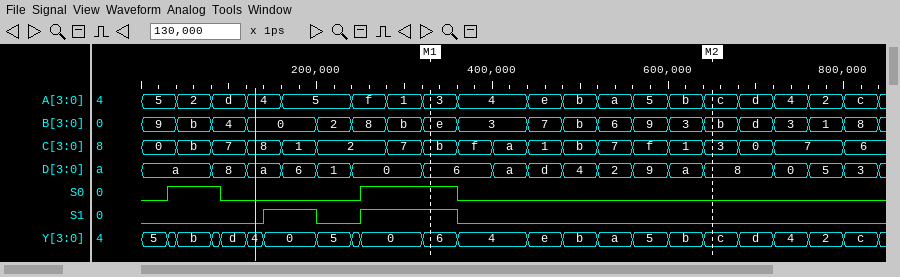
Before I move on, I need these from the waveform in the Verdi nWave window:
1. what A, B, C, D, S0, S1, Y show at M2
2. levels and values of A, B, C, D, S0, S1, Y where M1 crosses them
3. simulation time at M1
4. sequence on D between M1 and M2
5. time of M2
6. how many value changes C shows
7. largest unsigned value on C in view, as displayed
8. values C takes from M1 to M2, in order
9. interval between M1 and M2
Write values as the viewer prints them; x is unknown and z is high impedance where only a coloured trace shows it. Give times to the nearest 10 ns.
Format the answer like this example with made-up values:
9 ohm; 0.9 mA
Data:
A=c, B=b, C=3, D=8, S0=0, S1=0, Y=c; A=3, B=e, C=b, D=6, S0=1, S1=1, Y=6; 330 ns; 6, a, d, 4, 2, 9, a, 8; 650 ns; 18; f; b, f, a, 1, b, 7, f, 1, 3; 320 ns
